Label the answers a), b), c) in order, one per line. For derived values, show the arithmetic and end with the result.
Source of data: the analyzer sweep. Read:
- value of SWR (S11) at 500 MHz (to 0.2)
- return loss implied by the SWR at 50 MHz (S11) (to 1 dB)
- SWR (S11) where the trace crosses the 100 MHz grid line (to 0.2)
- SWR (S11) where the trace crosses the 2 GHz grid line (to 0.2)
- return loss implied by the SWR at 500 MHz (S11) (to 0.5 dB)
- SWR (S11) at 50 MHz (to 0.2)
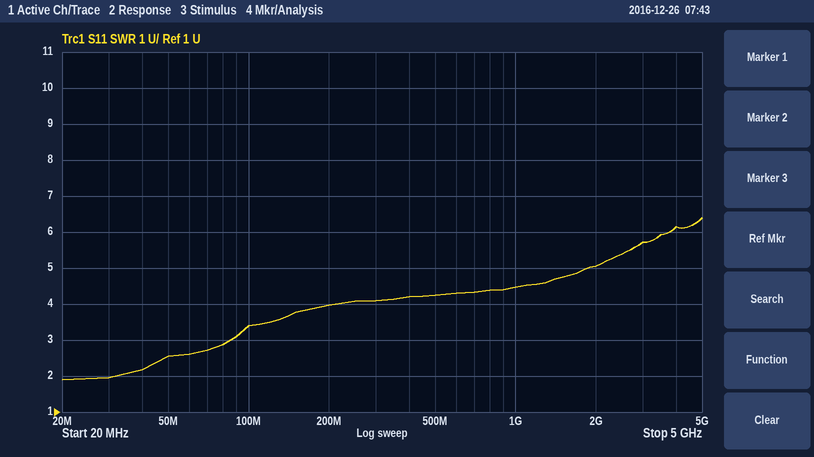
a) 4.2
b) −20 log10((2.6 − 1)/(2.6 + 1)) ≈ 7 dB
c) 3.4
d) 5.0
e) −20 log10((4.2 − 1)/(4.2 + 1)) ≈ 4.22 dB, so 4.0 dB to the nearest 0.5 dB
f) 2.6
